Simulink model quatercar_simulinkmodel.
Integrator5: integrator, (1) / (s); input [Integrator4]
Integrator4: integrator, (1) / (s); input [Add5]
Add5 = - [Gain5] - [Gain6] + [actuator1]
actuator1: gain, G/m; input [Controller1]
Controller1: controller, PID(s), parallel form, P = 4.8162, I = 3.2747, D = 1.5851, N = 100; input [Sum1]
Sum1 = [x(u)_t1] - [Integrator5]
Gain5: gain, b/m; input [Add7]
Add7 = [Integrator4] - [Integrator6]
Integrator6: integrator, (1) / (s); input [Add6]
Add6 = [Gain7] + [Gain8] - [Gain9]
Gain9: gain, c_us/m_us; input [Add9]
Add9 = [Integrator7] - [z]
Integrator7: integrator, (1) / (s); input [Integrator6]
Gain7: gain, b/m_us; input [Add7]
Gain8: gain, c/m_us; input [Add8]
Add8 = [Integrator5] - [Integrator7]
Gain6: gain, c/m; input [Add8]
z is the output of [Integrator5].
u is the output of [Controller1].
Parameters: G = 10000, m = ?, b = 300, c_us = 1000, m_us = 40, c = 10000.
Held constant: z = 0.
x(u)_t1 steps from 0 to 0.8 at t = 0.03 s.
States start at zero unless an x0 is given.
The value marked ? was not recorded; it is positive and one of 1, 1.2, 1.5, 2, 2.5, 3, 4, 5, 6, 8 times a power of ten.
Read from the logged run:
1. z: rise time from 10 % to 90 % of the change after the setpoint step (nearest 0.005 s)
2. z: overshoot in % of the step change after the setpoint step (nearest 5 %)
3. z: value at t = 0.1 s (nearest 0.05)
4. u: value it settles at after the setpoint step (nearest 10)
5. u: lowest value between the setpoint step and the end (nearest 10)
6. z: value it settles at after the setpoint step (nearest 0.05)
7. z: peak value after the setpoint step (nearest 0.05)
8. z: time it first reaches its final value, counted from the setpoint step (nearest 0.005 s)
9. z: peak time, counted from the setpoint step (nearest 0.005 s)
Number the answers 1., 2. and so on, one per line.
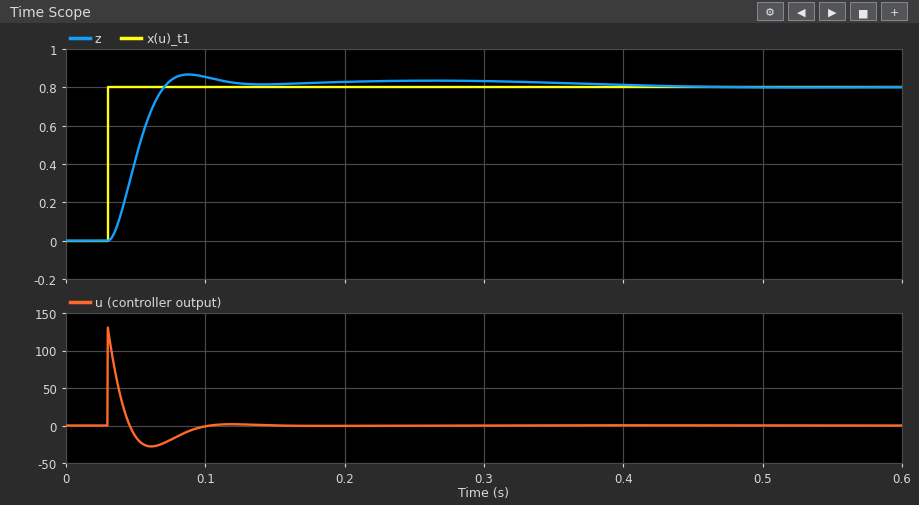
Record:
1. 0.025 s
2. 10 %
3. 0.85
4. 0
5. -30
6. 0.80
7. 0.85
8. 0.040 s
9. 0.060 s
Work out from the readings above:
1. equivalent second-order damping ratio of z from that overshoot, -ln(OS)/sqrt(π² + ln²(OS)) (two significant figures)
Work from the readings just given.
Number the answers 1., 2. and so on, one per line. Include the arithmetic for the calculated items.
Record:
1. ln(0.1) = -2.303; 2.303 / sqrt(9.870 + 5.302) = 0.59
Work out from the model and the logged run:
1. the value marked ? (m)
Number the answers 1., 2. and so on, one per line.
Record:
1. 300
